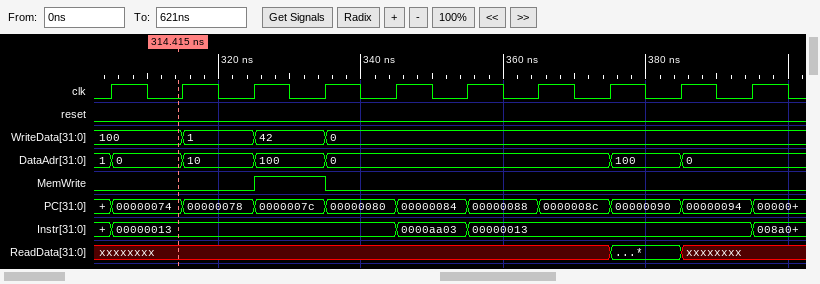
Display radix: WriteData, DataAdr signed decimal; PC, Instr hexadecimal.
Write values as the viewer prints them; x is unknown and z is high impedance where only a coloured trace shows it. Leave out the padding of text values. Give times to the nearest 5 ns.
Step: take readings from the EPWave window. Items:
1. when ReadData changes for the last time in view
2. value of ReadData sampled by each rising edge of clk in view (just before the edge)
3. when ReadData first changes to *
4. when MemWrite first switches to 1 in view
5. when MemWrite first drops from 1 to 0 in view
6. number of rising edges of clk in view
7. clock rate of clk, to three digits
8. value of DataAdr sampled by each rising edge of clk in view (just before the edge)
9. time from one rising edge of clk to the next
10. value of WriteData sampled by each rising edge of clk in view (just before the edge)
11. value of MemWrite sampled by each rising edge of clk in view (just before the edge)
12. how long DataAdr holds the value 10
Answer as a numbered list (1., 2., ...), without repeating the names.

1. 385 ns
2. xxxxxxxx, xxxxxxxx, xxxxxxxx, xxxxxxxx, xxxxxxxx, xxxxxxxx, xxxxxxxx, xxxxxxxx, *, xxxxxxxx
3. 375 ns
4. 325 ns
5. 335 ns
6. 10
7. 100 MHz
8. 1, 0, 10, 100, 0, 0, 0, 0, 100, 0
9. 10 ns
10. 100, 100, 1, 42, 0, 0, 0, 0, 0, 0
11. 0 0 0 1 0 0 0 0 0 0
12. 10 ns
